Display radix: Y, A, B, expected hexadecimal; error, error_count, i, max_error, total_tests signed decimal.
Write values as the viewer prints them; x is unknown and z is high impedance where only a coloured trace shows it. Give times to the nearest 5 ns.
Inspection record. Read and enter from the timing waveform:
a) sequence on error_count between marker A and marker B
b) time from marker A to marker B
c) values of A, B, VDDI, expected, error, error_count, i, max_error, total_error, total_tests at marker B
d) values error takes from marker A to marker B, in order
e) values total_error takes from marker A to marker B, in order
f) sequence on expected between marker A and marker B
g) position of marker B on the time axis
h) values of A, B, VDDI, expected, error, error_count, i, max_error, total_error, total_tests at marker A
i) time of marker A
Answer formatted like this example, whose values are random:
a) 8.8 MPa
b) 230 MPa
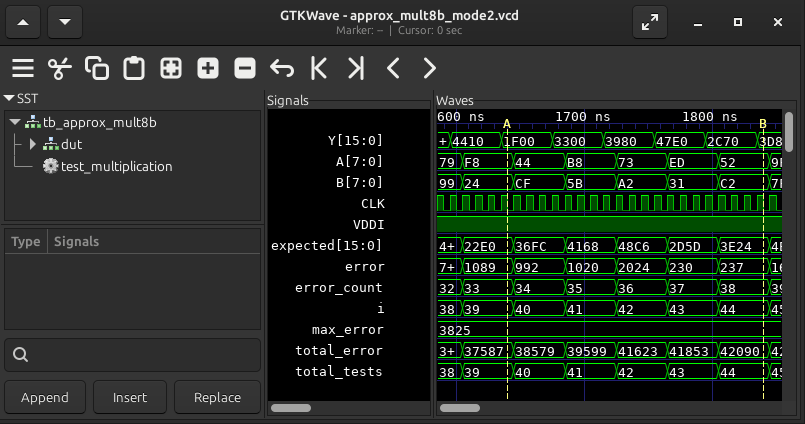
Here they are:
a) 33, 34, 35, 36, 37, 38
b) 200 ns
c) A=52, B=C2, VDDI=1, expected=3E24, error=237, error_count=38, i=44, max_error=3825, total_error=42090, total_tests=44
d) 1089, 992, 1020, 2024, 230, 237
e) 37587, 38579, 39599, 41623, 41853, 42090
f) 22E0, 36FC, 4168, 48C6, 2D5D, 3E24
g) 1840 ns
h) A=F8, B=24, VDDI=1, expected=22E0, error=1089, error_count=33, i=39, max_error=3825, total_error=37587, total_tests=39
i) 1640 ns
